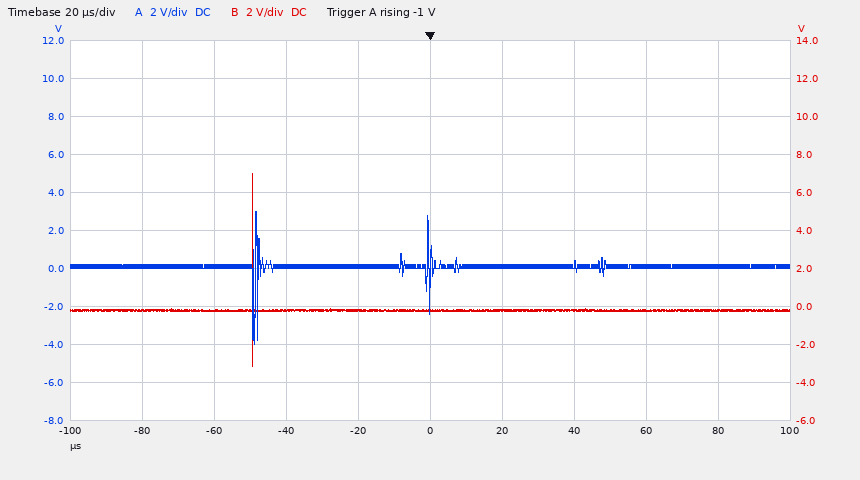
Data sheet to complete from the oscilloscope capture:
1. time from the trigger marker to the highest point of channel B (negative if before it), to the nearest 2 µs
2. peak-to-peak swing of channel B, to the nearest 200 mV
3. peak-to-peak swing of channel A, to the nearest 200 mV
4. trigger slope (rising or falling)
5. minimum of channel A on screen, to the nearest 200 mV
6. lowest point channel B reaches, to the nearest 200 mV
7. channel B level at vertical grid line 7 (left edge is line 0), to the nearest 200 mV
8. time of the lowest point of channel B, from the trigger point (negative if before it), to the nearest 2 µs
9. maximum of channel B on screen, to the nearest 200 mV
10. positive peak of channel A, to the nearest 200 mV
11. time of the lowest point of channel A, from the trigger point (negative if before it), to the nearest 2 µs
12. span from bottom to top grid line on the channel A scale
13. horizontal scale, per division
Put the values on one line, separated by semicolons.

-50 µs; 10.2 V; 7.0 V; rising; -4.0 V; -3.2 V; -200 mV; -50 µs; 7.0 V; 3.0 V; -48 µs; 20 V; 20 µs
